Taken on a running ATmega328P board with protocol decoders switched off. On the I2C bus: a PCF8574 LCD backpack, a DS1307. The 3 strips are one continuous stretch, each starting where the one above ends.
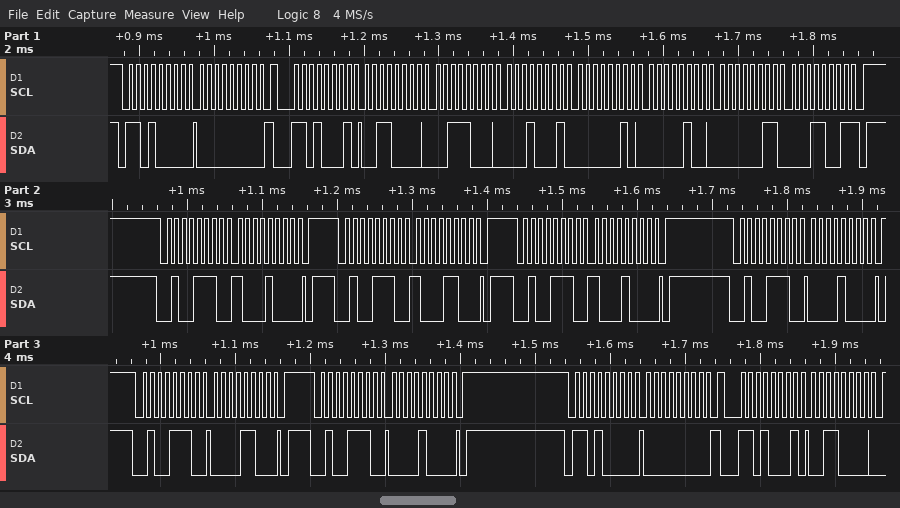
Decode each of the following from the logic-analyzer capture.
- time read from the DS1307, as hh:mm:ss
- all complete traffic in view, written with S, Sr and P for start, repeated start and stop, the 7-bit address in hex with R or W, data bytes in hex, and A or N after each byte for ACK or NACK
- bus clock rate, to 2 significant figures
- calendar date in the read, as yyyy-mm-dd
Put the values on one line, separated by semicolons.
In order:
11:38:30; S 68W A 00 A Sr 68R A 30 A 38 A 11 A 02 A 04 A 03 A 19 N P S 27W A 88 A P S 27W A 8C A P S 27W A 88 A P S 27W A 08 A P S 27W A 0C A P S 27W A 08 A P S 68W A 00 A Sr 68R A 30 A; 100 kHz; 2019-03-04
